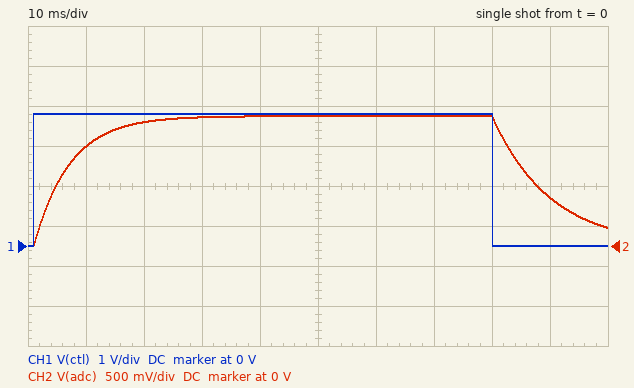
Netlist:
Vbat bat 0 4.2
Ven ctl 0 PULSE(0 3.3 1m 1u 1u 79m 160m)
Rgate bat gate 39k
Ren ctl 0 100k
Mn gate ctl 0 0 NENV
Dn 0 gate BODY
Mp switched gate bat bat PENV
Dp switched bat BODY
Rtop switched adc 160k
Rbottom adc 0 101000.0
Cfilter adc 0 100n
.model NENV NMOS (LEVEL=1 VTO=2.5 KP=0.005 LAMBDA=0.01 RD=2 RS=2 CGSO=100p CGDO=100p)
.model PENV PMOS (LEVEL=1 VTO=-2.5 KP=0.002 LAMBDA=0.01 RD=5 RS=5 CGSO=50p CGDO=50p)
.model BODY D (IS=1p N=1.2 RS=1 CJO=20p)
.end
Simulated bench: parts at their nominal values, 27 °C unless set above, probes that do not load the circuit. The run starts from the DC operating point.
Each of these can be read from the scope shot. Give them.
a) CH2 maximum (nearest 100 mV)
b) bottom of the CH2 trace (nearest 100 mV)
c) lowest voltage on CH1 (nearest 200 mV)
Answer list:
1.6 V
0 V
0 V
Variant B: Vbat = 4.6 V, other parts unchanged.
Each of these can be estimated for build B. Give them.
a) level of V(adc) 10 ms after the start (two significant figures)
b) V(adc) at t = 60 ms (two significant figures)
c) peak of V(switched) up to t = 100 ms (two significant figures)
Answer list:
1.4 V
1.8 V
4.6 V
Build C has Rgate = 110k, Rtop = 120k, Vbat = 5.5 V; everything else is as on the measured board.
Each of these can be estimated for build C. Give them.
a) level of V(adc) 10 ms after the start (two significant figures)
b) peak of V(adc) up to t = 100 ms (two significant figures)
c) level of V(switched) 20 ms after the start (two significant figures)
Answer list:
2.0 V
2.5 V
5.5 V
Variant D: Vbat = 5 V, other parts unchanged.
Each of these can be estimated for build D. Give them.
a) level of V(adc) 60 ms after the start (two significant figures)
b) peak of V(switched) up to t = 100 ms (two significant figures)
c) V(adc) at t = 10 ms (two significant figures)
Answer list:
1.9 V
5.0 V
1.5 V
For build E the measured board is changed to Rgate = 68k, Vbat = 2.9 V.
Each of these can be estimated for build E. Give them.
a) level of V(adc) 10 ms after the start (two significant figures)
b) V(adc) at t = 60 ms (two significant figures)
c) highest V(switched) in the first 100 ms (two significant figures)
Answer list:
850 mV
1.1 V
2.9 V
